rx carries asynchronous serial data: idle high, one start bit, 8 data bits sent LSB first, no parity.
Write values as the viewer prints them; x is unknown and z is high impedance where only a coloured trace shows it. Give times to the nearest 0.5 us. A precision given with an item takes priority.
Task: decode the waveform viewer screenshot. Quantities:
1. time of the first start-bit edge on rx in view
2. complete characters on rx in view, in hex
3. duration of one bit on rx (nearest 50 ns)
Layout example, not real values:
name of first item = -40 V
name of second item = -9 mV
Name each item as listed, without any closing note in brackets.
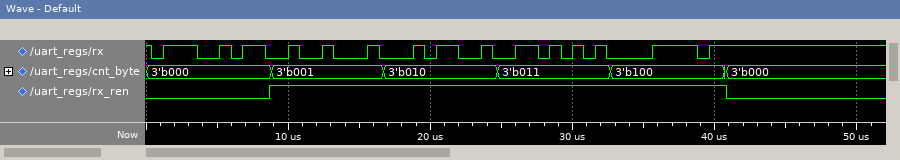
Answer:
time of the first start-bit edge on rx in view = 0.5 us
complete characters on rx in view, in hex = A7, 12, 34, 56, 78
duration of one bit on rx = 800 ns
